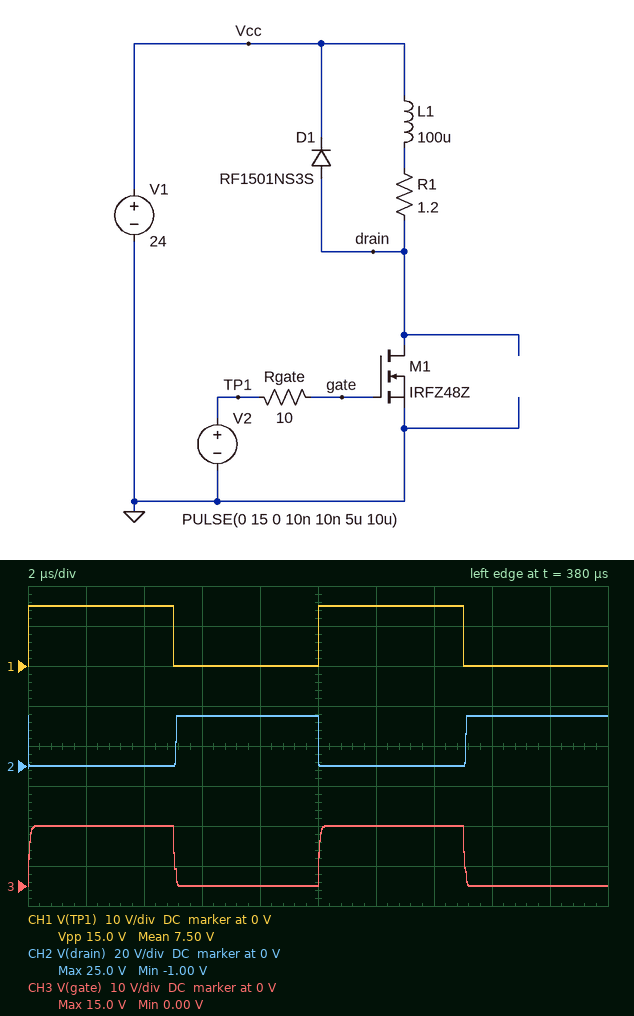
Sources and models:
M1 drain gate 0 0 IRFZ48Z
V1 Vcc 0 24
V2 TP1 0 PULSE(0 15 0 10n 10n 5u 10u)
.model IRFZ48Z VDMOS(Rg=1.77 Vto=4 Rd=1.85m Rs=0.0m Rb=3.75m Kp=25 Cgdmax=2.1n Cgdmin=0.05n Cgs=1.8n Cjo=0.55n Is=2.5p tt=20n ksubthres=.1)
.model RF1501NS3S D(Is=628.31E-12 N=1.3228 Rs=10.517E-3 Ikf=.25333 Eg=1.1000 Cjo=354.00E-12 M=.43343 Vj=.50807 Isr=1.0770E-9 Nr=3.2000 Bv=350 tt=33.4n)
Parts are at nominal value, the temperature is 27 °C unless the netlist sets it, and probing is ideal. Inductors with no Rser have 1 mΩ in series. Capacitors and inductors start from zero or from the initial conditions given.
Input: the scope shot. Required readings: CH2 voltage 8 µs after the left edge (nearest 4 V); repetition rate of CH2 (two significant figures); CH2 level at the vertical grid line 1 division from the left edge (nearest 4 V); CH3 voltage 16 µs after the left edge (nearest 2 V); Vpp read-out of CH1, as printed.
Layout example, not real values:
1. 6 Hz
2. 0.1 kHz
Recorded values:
1. 24 V
2. 100 kHz
3. 0 V
4. 0 V
5. 15.0 V
